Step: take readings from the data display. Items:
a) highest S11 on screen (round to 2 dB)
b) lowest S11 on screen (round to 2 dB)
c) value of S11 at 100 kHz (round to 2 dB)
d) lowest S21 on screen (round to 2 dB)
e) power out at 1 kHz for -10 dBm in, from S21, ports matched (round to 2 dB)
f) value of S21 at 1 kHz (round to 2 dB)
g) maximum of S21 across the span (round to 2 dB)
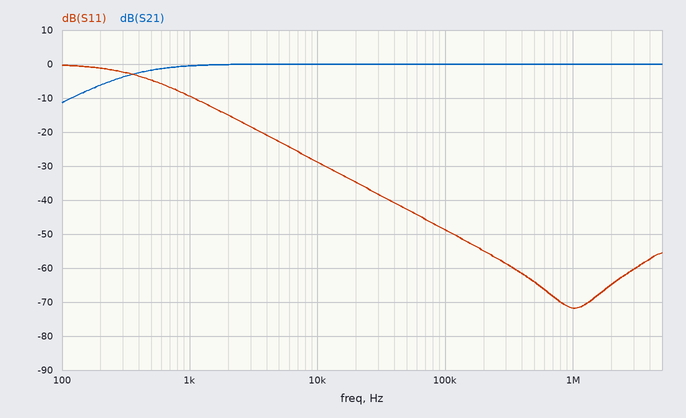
0 dB
-72 dB
-48 dB
-12 dB
-10 dBm
0 dB
0 dB
